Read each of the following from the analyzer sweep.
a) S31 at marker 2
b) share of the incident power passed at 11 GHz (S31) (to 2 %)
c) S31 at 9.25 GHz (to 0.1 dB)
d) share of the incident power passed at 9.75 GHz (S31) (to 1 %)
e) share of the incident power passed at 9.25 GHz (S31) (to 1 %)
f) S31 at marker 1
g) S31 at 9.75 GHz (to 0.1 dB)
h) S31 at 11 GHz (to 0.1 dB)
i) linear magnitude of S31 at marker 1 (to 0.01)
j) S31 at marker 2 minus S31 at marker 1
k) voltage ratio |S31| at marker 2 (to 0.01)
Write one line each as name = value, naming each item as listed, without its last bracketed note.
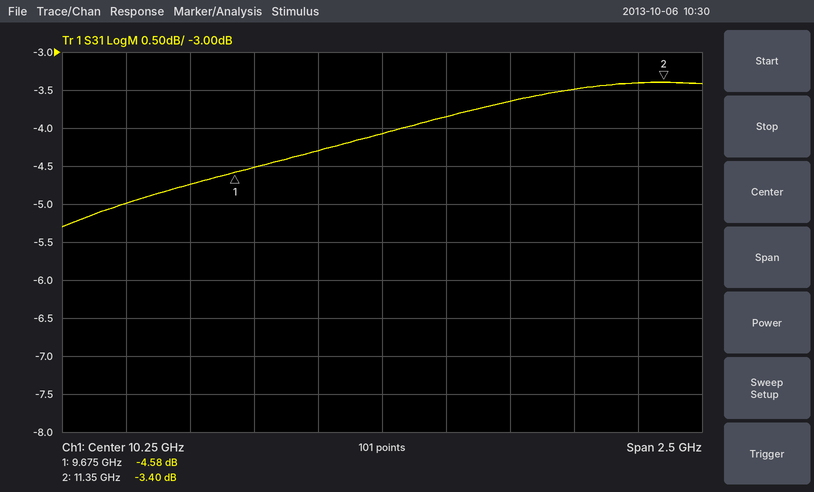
S31 at marker 2 = -3.40 dB
share of the incident power passed at 11 GHz (S31) = 44 %
S31 at 9.25 GHz = -5.0 dB
share of the incident power passed at 9.75 GHz (S31) = 35 %
share of the incident power passed at 9.25 GHz (S31) = 32 %
S31 at marker 1 = -4.58 dB
S31 at 9.75 GHz = -4.5 dB
S31 at 11 GHz = -3.5 dB
linear magnitude of S31 at marker 1 = 0.59
S31 at marker 2 minus S31 at marker 1 = 1.18 dB
voltage ratio |S31| at marker 2 = 0.68
